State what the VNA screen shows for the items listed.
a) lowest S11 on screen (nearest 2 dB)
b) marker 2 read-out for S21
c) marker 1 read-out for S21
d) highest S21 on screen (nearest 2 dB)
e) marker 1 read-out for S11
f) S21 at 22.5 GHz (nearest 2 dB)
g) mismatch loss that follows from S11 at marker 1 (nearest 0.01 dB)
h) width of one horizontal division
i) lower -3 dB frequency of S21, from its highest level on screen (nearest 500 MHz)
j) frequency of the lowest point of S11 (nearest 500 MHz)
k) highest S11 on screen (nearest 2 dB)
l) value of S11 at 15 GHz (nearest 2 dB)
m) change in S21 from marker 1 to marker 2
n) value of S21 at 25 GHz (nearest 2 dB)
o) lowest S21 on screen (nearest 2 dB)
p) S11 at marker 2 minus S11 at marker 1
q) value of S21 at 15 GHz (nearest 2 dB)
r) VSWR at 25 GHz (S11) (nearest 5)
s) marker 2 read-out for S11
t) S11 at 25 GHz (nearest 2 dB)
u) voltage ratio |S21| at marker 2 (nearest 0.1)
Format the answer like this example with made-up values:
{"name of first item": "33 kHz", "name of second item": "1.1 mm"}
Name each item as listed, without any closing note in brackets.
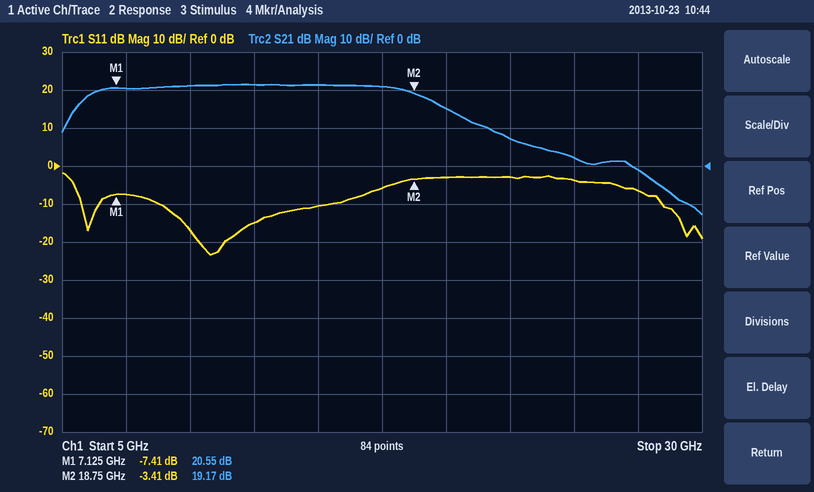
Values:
{"lowest S11 on screen": "-24 dB", "marker 2 read-out for S21": "19.17 dB", "marker 1 read-out for S21": "20.55 dB", "highest S21 on screen": "22 dB", "marker 1 read-out for S11": "-7.41 dB", "S21 at 22.5 GHz": "8 dB", "mismatch loss that follows from S11 at marker 1": "0.87 dB", "width of one horizontal division": "2.5 GHz", "lower -3 dB frequency of S21, from its highest level on screen": "6.0 GHz", "frequency of the lowest point of S11": "11.0 GHz", "highest S11 on screen": "-2 dB", "value of S11 at 15 GHz": "-10 dB", "change in S21 from marker 1 to marker 2": "-1.38 dB", "value of S21 at 25 GHz": "2 dB", "lowest S21 on screen": "-12 dB", "S11 at marker 2 minus S11 at marker 1": "4.00 dB", "value of S21 at 15 GHz": "22 dB", "VSWR at 25 GHz (S11)": "5", "marker 2 read-out for S11": "-3.41 dB", "S11 at 25 GHz": "-4 dB", "voltage ratio |S21| at marker 2": "9.1"}
